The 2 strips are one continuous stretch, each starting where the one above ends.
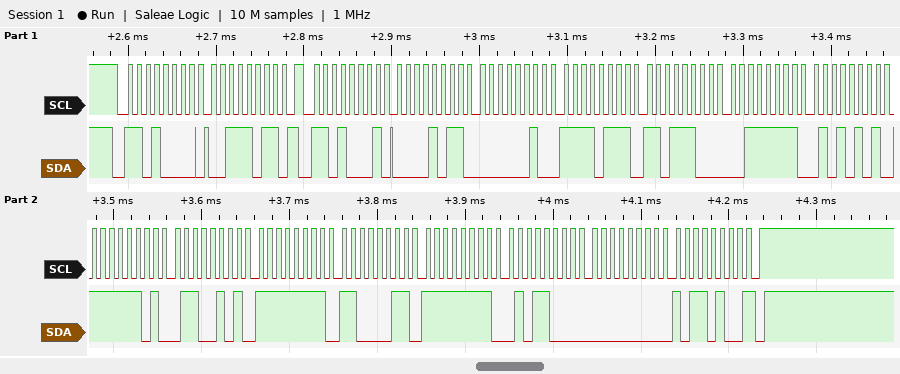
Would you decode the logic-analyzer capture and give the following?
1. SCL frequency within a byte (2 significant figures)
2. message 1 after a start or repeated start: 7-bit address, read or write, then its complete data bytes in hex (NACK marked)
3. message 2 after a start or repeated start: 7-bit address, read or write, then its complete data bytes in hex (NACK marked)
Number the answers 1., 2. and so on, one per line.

1. 100 kHz
2. 0x68 write: 3B
3. 0x68 read: 0B 02 F7 DC 3F 55 FD 65 FF C3 FF 58 00 B4 NACK
